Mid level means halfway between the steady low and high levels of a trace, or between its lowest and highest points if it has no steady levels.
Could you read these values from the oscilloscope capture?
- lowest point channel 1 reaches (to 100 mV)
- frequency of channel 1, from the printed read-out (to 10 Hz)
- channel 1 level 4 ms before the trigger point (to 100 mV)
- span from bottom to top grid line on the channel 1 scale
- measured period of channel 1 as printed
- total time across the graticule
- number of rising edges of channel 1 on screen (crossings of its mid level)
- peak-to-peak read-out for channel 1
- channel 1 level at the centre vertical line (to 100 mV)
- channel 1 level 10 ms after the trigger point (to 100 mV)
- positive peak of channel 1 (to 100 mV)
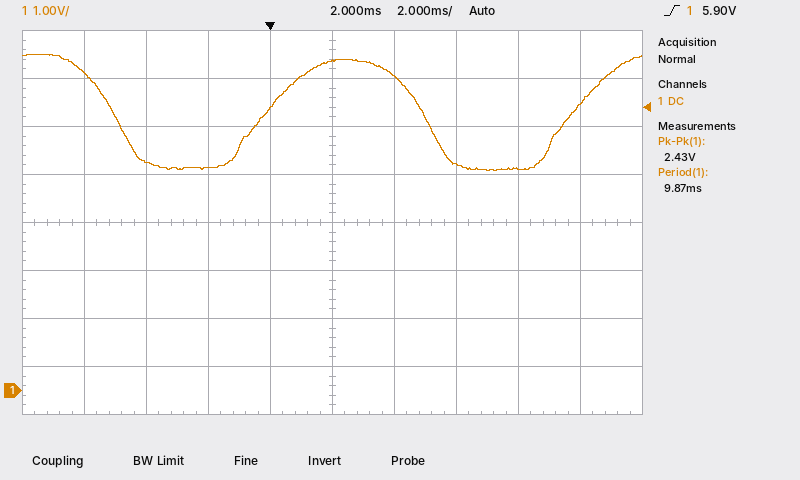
4.6 V
100 Hz
4.8 V
8 V
9.87 ms
20 ms
2
2.43 V
6.9 V
6.0 V
7.0 V
